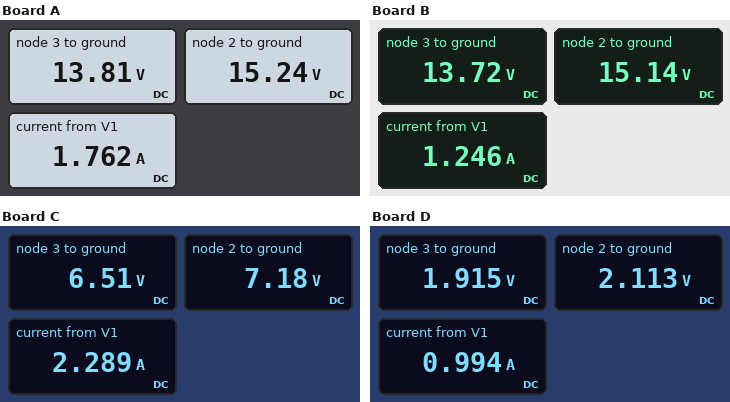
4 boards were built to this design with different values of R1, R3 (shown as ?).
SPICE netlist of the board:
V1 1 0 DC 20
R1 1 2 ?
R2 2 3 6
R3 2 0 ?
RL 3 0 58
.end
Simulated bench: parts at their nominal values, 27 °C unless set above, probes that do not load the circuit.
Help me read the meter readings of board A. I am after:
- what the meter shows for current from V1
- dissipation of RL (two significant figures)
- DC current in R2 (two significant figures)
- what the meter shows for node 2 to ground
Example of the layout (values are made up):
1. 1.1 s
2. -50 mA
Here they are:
1. 1.762 A
2. 3.3 W
3. 240 mA
4. 15.24 V
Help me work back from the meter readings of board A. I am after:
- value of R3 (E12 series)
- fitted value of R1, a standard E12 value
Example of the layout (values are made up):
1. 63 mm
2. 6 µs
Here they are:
1. 10 Ω
2. 2.7 Ω
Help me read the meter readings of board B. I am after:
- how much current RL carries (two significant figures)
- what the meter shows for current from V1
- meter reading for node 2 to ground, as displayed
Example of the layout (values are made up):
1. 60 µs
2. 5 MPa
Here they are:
1. 240 mA
2. 1.246 A
3. 15.14 V
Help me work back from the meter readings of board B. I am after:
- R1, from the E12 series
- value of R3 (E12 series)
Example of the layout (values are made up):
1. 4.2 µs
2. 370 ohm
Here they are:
1. 3.9 Ω
2. 15 Ω
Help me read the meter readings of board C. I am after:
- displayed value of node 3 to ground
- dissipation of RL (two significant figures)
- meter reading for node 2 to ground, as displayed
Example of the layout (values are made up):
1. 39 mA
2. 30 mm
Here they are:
1. 6.51 V
2. 730 mW
3. 7.18 V
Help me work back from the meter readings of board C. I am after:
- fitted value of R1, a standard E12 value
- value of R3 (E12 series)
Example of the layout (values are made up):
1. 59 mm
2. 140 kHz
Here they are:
1. 5.6 Ω
2. 3.3 Ω
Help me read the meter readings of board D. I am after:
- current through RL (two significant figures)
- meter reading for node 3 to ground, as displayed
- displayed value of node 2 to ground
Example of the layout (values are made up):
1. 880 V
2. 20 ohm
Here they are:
1. 33 mA
2. 1.915 V
3. 2.113 V
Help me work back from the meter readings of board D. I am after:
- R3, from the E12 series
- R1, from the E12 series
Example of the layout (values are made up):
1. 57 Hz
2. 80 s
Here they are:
1. 2.2 Ω
2. 18 Ω
